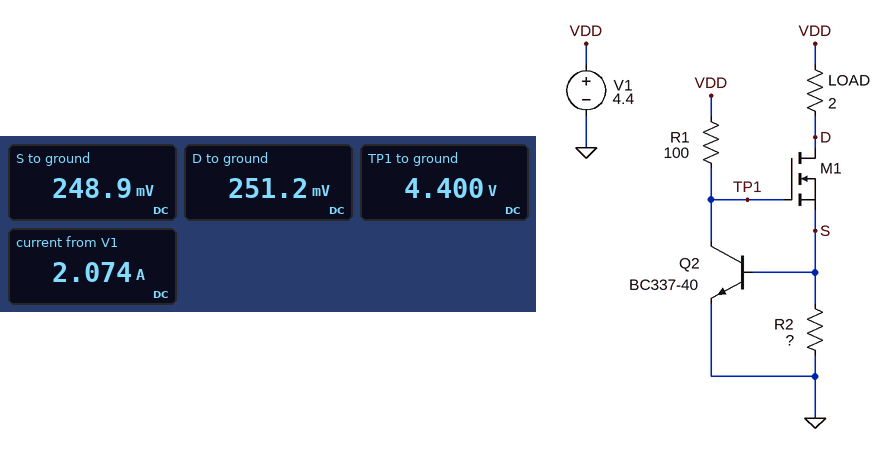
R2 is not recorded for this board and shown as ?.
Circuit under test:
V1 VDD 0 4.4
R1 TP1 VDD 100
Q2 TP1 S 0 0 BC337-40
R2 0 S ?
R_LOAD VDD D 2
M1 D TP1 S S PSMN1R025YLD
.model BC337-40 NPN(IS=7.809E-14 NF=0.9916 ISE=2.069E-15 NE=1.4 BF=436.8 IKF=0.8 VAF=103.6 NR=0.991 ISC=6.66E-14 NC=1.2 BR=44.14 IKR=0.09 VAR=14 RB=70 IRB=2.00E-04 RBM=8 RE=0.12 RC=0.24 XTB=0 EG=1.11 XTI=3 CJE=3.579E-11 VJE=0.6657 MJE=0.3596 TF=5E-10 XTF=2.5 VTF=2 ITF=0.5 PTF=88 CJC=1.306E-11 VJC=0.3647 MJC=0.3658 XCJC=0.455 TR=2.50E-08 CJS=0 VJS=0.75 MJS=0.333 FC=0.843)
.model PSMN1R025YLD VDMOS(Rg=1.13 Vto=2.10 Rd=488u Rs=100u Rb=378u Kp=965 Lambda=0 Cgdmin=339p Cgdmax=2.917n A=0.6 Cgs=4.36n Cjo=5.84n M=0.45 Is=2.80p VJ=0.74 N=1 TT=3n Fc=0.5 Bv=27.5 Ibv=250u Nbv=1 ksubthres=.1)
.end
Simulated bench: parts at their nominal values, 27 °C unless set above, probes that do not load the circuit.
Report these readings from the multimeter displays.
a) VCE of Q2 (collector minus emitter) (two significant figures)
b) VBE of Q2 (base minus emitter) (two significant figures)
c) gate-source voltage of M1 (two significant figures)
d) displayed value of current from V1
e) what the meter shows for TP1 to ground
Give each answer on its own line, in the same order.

4.4 V
250 mV
4.2 V
2.074 A
4.400 V
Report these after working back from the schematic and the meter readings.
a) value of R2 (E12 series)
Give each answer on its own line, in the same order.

0.12 Ω
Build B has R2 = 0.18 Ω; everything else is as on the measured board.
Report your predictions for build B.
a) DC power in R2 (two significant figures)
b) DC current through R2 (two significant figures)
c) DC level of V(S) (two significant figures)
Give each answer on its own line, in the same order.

730 mW
2.0 A
360 mV
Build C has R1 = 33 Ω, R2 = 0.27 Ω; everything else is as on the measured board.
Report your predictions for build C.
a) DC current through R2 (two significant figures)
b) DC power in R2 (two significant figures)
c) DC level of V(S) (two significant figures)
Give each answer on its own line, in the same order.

1.9 A
1.0 W
520 mV
